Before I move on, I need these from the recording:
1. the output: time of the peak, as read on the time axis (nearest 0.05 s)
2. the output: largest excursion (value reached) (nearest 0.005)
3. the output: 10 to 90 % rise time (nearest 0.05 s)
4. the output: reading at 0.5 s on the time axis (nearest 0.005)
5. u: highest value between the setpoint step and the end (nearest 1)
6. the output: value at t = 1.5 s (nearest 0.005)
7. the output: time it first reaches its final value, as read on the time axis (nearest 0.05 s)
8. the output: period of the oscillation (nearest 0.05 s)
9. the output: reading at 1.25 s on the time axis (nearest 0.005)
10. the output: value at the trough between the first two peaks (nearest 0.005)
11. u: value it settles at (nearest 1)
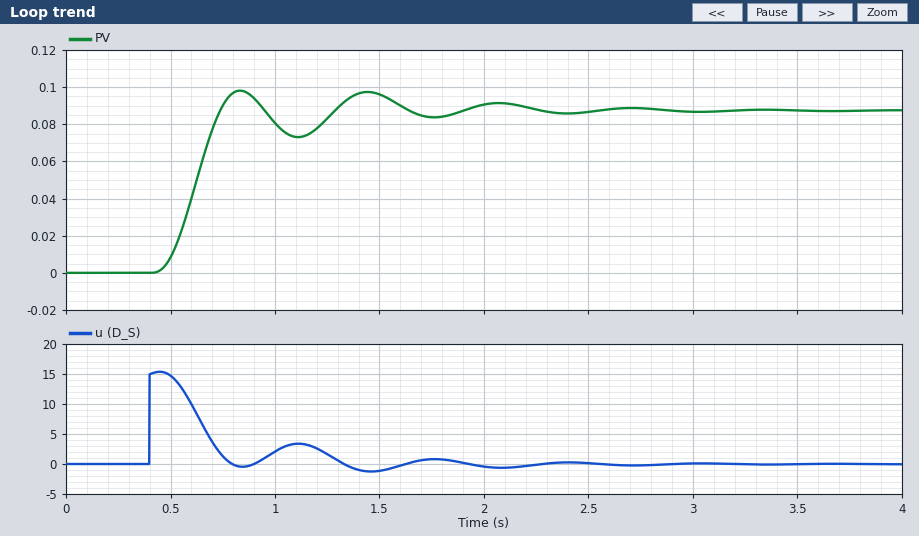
0.85 s
0.100
0.20 s
0.010
15
0.095
0.75 s
0.60 s
0.085
0.075
0
